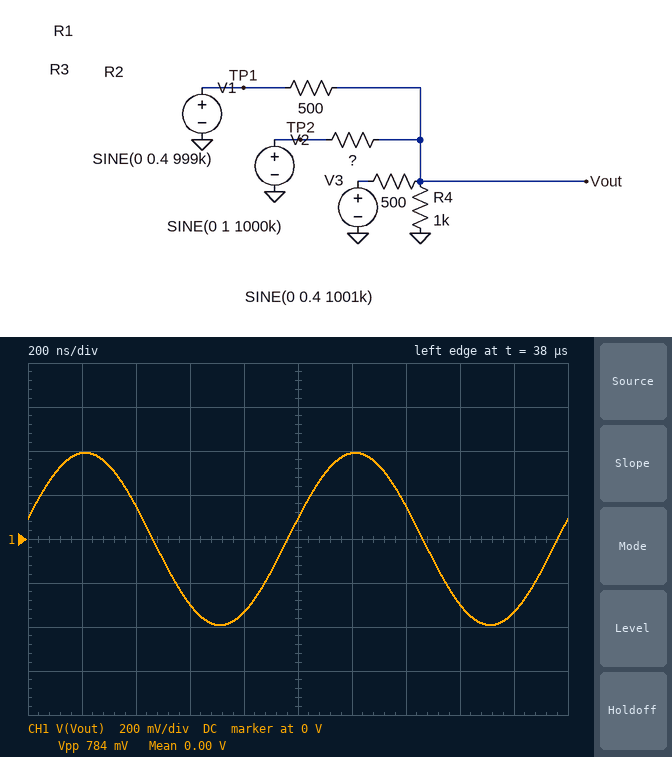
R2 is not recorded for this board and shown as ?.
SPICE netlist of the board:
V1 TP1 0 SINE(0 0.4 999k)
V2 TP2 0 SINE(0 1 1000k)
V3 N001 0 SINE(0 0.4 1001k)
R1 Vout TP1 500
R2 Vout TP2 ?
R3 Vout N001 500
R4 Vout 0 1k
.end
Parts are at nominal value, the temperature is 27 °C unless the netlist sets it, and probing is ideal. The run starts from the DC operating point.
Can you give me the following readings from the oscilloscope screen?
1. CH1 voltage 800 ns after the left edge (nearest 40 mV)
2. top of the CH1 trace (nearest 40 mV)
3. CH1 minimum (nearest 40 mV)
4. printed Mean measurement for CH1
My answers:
-320 mV
400 mV
-400 mV
0.00 V
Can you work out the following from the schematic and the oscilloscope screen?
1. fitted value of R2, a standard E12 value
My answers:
1.5 kΩ
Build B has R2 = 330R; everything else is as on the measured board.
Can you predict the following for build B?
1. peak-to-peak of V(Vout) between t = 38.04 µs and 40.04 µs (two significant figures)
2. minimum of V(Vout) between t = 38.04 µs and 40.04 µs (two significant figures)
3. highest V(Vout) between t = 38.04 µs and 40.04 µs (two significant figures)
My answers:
1.1 V
-570 mV
570 mV
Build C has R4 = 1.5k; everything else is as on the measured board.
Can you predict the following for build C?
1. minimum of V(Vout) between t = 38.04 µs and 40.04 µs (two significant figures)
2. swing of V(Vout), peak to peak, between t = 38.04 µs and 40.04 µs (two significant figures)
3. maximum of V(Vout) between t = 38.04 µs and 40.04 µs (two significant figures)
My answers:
-420 mV
830 mV
420 mV
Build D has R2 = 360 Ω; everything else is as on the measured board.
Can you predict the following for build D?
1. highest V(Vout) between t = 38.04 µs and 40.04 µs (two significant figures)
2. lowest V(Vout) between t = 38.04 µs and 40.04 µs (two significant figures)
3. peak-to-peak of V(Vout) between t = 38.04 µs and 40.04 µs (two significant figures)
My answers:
560 mV
-560 mV
1.1 V
